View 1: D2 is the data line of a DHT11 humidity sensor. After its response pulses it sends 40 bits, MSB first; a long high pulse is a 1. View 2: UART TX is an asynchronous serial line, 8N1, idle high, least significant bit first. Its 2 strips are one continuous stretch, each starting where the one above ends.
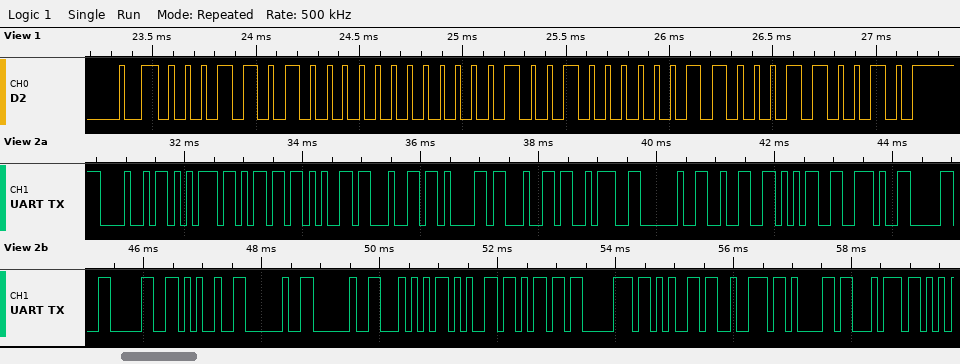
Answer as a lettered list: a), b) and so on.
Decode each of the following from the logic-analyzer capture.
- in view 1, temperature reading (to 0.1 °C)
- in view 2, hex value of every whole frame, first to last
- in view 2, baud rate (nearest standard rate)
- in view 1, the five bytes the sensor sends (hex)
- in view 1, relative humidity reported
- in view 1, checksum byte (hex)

a) 18.6 °C
b) 0x48 0x75 0x6D 0x65 0x64 0x61 0x64 0x3A 0x20 0x32 0x35 0x2E 0x30 0x30 0x25 0x20 0x20 0x54 0x65 0x6D 0x70 0x65 0x72 0x61 0x74
c) 9600 baud
d) 1A 00 12 06 32
e) 26 %
f) 0x32
